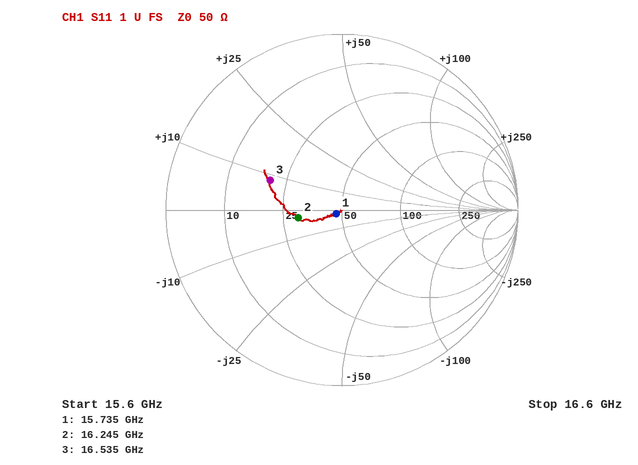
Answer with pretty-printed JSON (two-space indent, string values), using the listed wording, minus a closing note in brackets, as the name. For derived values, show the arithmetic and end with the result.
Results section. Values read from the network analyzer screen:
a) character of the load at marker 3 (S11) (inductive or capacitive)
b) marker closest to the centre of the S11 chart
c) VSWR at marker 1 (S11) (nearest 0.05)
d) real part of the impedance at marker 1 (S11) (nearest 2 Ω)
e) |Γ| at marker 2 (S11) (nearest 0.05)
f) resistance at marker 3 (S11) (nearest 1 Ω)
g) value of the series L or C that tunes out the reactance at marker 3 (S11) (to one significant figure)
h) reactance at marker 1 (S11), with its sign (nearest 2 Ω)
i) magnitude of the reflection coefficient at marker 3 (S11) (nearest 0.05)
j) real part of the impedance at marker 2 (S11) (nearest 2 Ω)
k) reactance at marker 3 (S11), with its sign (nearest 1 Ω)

{
  "character of the load at marker 3 (S11)": "inductive",
  "marker closest to the centre of the S11 chart": "marker 1",
  "VSWR at marker 1 (S11)": "1.10",
  "real part of the impedance at marker 1 (S11)": "46 Ω",
  "|Γ| at marker 2 (S11)": "0.25",
  "resistance at marker 3 (S11)": "20 Ω",
  "value of the series L or C that tunes out the reactance at marker 3 (S11)": "C = 1/(2π × 16.535 GHz × 8 Ω) ≈ 1 pF",
  "reactance at marker 1 (S11), with its sign": "-2 Ω",
  "magnitude of the reflection coefficient at marker 3 (S11)": "0.45",
  "real part of the impedance at marker 2 (S11)": "30 Ω",
  "reactance at marker 3 (S11), with its sign": "+8 Ω"
}
